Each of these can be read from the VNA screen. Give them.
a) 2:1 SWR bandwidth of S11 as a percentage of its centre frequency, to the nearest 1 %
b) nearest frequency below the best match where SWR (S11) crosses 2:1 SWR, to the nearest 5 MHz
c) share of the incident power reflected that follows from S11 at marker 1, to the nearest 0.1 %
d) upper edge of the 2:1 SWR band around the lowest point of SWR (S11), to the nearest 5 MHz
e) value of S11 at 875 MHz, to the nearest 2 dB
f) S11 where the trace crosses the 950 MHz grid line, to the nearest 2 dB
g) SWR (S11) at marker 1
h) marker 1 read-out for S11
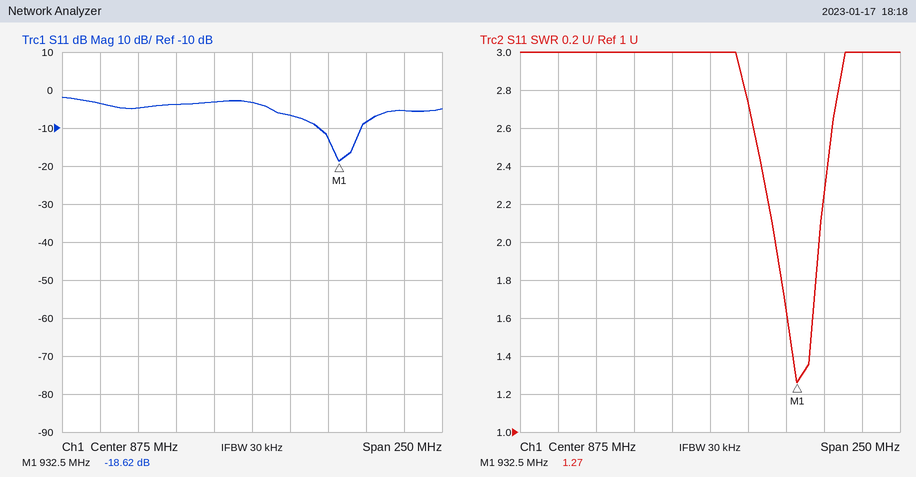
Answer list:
3 %
920 MHz
1.4 %
945 MHz
-4 dB
-8 dB
1.27
-18.62 dB
